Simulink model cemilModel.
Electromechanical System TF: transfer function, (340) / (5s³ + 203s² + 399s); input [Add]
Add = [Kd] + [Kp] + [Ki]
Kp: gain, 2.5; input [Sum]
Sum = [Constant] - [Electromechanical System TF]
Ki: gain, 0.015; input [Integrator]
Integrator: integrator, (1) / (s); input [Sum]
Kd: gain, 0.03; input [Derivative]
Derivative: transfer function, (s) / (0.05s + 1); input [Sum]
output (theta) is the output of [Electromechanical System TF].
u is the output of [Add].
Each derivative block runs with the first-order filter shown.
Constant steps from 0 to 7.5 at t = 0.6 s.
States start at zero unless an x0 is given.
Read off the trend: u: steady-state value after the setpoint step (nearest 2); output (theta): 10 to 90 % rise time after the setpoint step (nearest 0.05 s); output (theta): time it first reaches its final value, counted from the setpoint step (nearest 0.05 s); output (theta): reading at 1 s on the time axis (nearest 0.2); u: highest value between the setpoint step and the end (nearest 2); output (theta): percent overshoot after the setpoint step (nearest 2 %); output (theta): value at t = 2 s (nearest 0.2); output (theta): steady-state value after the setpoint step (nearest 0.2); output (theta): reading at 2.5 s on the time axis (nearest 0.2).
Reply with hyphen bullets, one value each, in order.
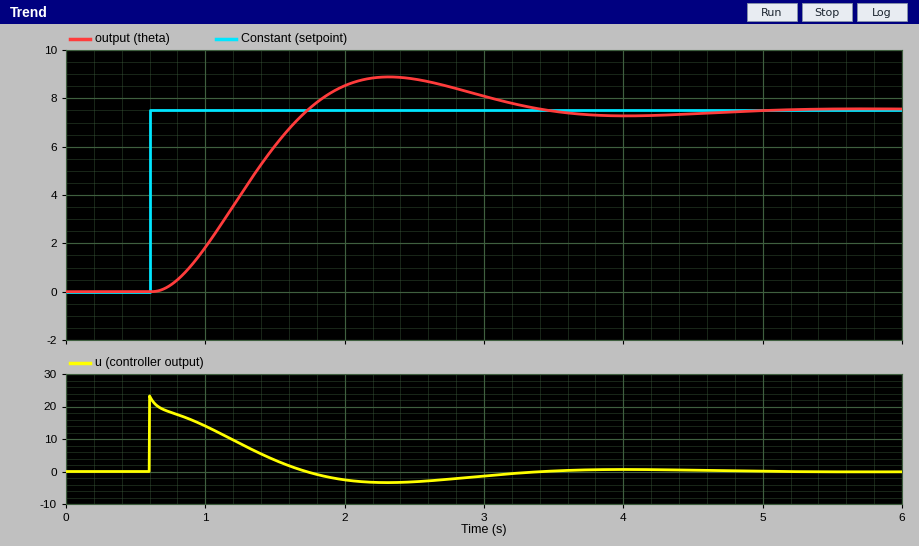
- 0
- 0.75 s
- 1.15 s
- 1.8
- 24
- 18 %
- 8.6
- 7.6
- 8.8
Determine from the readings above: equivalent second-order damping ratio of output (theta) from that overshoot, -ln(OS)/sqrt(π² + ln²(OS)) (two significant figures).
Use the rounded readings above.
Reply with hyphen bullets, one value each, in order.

- 0.48
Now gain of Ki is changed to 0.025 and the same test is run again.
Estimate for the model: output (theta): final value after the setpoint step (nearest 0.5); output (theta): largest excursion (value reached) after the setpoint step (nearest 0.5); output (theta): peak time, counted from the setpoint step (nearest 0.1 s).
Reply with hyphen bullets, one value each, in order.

- 7.5
- 9.0
- 1.7 s
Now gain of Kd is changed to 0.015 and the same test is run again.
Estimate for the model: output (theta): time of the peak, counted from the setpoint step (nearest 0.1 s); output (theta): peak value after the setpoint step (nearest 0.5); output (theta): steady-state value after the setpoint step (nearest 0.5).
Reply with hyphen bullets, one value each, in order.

- 1.7 s
- 9.0
- 7.5
